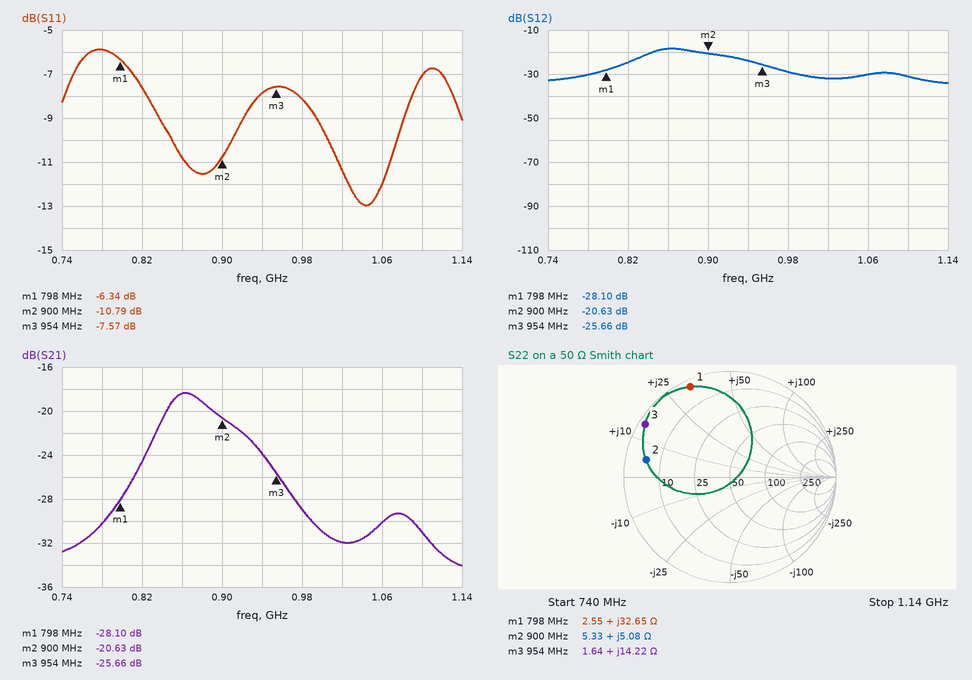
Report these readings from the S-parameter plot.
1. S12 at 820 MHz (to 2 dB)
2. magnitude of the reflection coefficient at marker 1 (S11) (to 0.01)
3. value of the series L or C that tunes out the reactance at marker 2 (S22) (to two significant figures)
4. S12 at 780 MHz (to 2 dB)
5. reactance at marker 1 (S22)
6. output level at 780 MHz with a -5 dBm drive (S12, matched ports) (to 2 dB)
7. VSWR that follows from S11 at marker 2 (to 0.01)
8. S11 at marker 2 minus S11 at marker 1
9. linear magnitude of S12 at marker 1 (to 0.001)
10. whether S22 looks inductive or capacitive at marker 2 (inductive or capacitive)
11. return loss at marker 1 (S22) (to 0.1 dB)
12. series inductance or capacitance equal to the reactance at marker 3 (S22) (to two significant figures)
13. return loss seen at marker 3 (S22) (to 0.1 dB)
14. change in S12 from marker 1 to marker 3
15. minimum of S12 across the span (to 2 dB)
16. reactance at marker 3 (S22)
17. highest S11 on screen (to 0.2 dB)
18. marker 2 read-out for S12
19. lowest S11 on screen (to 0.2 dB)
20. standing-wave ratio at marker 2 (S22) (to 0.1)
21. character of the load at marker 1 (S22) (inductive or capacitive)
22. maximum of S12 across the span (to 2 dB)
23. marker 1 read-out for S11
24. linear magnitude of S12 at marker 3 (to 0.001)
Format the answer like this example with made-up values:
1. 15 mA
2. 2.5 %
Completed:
1. -24 dB
2. 0.48
3. 35 pF
4. -30 dB
5. +32.65 Ω
6. -36 dBm
7. 1.81
8. -4.45 dB
9. 0.039
10. inductive
11. 0.6 dB
12. 2.4 nH
13. 0.5 dB
14. 2.44 dB
15. -34 dB
16. +14.22 Ω
17. -5.8 dB
18. -20.63 dB
19. -13.0 dB
20. 9.5
21. inductive
22. -18 dB
23. -6.34 dB
24. 0.052
